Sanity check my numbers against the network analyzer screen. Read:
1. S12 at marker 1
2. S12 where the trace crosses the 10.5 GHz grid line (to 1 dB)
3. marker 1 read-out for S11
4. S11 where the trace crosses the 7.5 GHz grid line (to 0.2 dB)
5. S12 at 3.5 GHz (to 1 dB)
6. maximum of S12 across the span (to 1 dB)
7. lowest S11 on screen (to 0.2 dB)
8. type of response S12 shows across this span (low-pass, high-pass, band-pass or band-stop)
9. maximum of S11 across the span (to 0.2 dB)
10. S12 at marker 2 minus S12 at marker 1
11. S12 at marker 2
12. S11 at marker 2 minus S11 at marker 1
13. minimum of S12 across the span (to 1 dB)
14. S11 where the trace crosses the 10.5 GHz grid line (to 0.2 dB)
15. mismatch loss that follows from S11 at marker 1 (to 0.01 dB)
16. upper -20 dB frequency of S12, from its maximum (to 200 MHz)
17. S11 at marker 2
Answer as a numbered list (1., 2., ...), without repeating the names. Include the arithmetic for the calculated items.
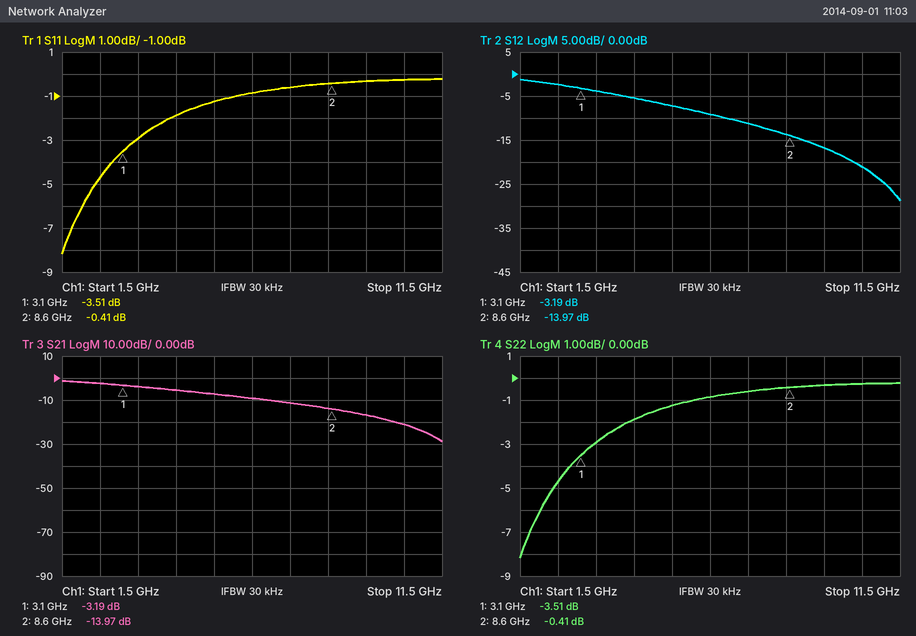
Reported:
1. -3.19 dB
2. -21 dB
3. -3.51 dB
4. -0.6 dB
5. -4 dB
6. -1 dB
7. -8.2 dB
8. low-pass
9. -0.2 dB
10. -13.97 − (-3.19) = -10.78 dB
11. -13.97 dB
12. -0.41 − (-3.51) = 3.10 dB
13. -29 dB
14. -0.2 dB
15. −10 log10(1 − 10^(-3.51/10)) ≈ 2.56 dB
16. 10.6 GHz
17. -0.41 dB
